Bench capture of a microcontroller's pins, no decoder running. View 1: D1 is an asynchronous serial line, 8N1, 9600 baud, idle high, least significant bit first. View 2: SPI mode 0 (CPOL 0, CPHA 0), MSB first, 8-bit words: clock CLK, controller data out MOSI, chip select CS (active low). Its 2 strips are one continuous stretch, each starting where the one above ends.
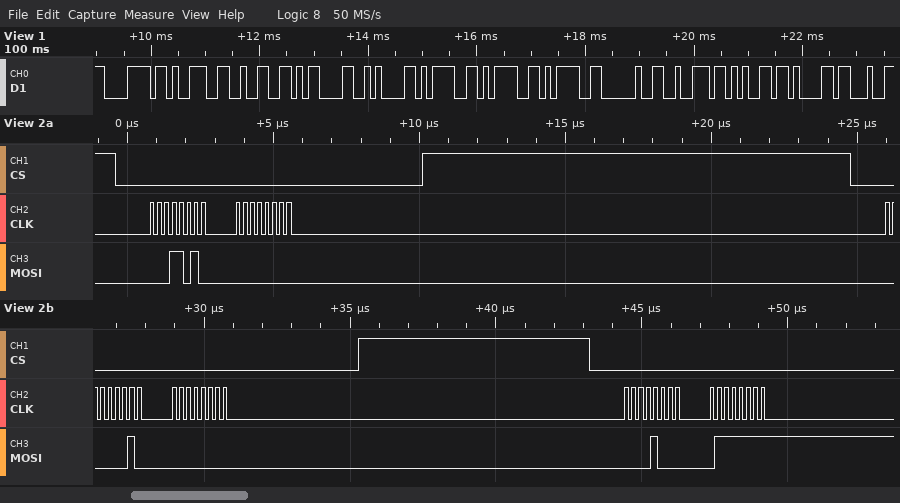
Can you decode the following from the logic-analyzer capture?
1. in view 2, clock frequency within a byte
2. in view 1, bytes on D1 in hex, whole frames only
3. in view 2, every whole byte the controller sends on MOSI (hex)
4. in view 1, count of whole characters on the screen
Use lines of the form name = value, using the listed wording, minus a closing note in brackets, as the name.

in view 2, clock frequency within a byte = 4 MHz
in view 1, bytes on D1 in hex, whole frames only = 78 39 32 0D 0A 3D 3D 3D 20 72 65 61
in view 2, every whole byte the controller sends on MOSI = 1A 00 02 00 08 7F
in view 1, count of whole characters on the screen = 12
